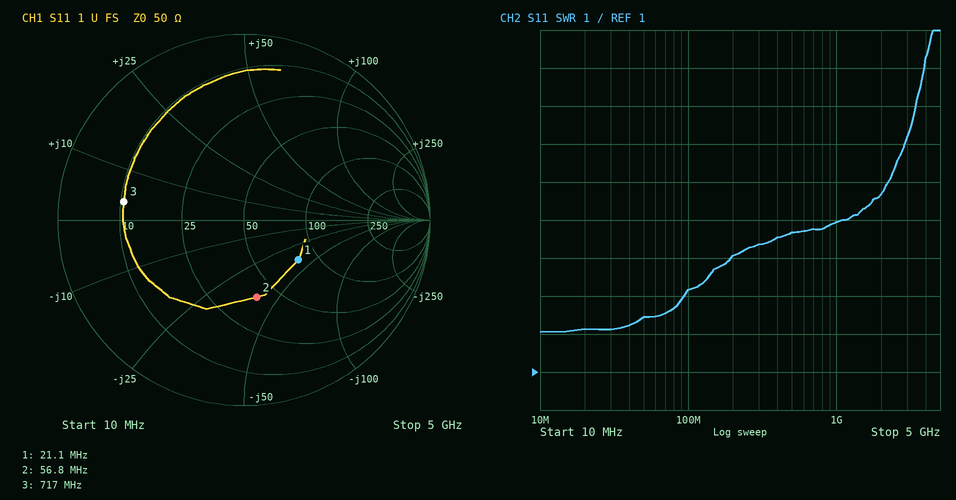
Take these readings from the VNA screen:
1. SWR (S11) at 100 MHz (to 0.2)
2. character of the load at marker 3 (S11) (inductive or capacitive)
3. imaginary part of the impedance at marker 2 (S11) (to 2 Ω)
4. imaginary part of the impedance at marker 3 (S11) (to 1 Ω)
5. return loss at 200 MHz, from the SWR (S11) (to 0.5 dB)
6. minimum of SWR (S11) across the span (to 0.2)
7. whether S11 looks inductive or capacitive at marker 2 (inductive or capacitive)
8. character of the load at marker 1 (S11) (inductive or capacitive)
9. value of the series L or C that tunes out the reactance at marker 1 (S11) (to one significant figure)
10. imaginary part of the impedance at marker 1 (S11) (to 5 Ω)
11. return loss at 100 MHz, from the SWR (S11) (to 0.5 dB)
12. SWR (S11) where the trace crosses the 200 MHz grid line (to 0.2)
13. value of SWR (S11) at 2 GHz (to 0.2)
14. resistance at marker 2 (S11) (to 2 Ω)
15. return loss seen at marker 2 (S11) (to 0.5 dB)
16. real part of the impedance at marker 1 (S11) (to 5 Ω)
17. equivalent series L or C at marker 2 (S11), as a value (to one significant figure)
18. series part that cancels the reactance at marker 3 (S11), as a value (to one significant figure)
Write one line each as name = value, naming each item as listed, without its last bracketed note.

SWR (S11) at 100 MHz = 3.2
character of the load at marker 3 (S11) = inductive
imaginary part of the impedance at marker 2 (S11) = -40 Ω
imaginary part of the impedance at marker 3 (S11) = +4 Ω
return loss at 200 MHz, from the SWR (S11) = 4.5 dB
minimum of SWR (S11) across the span = 2.0
whether S11 looks inductive or capacitive at marker 2 = capacitive
character of the load at marker 1 (S11) = capacitive
value of the series L or C that tunes out the reactance at marker 1 (S11) = 300 nH
imaginary part of the impedance at marker 1 (S11) = -40 Ω
return loss at 100 MHz, from the SWR (S11) = 5.5 dB
SWR (S11) where the trace crosses the 200 MHz grid line = 4.0
value of SWR (S11) at 2 GHz = 5.6
resistance at marker 2 (S11) = 40 Ω
return loss seen at marker 2 (S11) = 7.5 dB
real part of the impedance at marker 1 (S11) = 80 Ω
equivalent series L or C at marker 2 (S11), as a value = 70 pF
series part that cancels the reactance at marker 3 (S11), as a value = 60 pF
